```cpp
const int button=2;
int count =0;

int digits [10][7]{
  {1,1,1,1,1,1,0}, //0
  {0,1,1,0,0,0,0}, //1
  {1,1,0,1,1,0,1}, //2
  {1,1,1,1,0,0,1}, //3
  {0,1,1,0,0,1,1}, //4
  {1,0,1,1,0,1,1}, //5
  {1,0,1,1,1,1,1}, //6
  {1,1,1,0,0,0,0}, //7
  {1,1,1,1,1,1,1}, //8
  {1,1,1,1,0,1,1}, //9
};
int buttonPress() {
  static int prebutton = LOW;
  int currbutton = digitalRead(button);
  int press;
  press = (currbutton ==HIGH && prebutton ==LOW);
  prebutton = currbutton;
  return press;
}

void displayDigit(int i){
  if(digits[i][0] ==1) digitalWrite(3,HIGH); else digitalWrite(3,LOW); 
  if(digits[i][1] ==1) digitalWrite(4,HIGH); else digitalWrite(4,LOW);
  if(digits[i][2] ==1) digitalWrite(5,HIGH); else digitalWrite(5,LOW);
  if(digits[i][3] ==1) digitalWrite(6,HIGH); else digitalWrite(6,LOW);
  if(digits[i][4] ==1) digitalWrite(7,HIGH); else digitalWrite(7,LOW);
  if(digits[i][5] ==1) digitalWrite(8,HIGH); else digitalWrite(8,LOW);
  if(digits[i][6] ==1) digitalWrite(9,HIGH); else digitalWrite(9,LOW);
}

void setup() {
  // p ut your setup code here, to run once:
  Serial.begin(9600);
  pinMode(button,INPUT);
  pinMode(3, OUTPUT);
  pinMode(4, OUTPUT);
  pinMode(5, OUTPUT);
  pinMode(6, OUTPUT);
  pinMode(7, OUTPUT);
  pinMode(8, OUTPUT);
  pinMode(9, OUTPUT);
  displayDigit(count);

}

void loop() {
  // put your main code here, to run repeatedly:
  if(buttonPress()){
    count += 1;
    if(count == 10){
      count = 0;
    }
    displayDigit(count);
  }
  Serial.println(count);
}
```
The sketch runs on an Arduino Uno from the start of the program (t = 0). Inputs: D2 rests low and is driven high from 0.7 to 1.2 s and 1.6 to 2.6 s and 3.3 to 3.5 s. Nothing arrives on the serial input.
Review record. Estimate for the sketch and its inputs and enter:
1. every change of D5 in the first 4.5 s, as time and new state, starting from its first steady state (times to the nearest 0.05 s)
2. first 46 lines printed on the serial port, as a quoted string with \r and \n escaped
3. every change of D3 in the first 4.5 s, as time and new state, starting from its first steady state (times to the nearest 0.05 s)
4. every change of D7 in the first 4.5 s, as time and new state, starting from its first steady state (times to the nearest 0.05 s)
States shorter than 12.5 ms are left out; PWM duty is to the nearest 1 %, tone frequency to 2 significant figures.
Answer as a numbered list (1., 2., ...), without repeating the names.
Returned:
1. 0 s high; 1.6 s low; 3.3 s high
2. "0\r\n0\r\n0\r\n0\r\n0\r\n0\r\n0\r\n0\r\n0\r\n0\r\n0\r\n0\r\n0\r\n0\r\n0\r\n0\r\n0\r\n0\r\n0\r\n0\r\n0\r\n0\r\n0\r\n0\r\n0\r\n0\r\n0\r\n0\r\n0\r\n0\r\n0\r\n0\r\n0\r\n0\r\n0\r\n0\r\n0\r\n0\r\n0\r\n0\r\n0\r\n0\r\n0\r\n0\r\n0\r\n0\r\n"
3. 0 s high; 0.7 s low; 1.6 s high
4. 0 s high; 0.7 s low; 1.6 s high; 3.3 s low
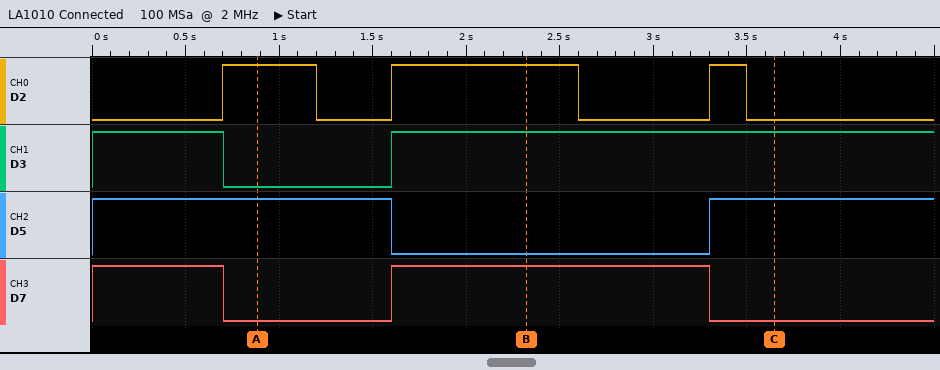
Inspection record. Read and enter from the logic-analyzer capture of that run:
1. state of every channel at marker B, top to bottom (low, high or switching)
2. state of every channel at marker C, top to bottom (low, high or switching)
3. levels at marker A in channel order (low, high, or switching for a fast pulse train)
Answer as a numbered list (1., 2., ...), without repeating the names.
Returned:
1. D2 high, D3 high, D5 low, D7 high
2. D2 low, D3 high, D5 high, D7 low
3. D2 high, D3 low, D5 high, D7 low
